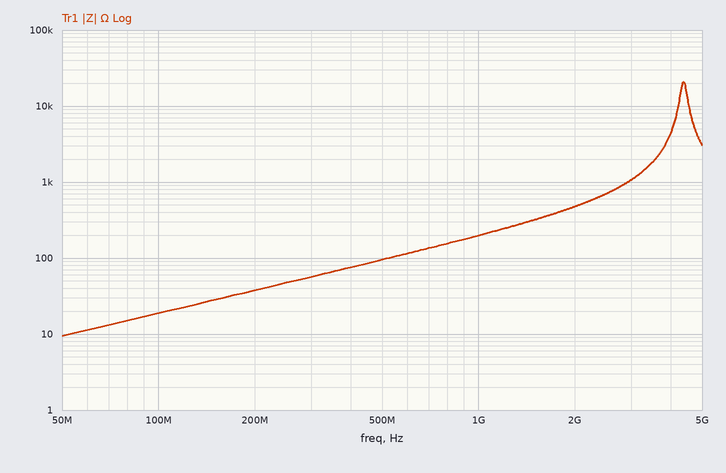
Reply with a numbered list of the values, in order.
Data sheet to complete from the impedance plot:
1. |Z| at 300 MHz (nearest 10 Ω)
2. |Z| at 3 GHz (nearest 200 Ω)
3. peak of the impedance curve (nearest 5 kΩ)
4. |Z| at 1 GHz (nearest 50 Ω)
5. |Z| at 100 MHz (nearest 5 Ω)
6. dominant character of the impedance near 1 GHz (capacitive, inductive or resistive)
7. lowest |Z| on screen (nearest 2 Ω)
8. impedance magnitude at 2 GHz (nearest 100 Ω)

1. 60 Ω
2. 1.0 kΩ
3. 20 kΩ
4. 200 Ω
5. 20 Ω
6. inductive
7. 10 Ω
8. 500 Ω
